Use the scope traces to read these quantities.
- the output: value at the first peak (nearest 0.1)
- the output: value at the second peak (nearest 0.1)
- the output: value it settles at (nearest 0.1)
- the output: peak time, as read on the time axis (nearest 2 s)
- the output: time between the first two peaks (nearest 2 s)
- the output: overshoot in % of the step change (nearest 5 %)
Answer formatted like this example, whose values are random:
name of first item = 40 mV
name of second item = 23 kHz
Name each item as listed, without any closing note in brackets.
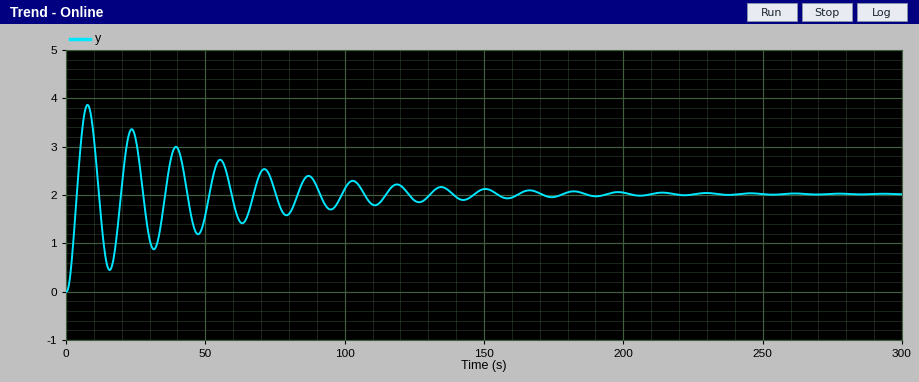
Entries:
the output: value at the first peak = 3.9
the output: value at the second peak = 3.4
the output: value it settles at = 2.0
the output: peak time, as read on the time axis = 8 s
the output: time between the first two peaks = 16 s
the output: overshoot in % of the step change = 90 %
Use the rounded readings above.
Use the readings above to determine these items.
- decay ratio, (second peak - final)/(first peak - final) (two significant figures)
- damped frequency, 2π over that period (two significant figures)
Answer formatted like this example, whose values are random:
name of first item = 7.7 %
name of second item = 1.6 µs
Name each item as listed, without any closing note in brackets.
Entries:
decay ratio, (second peak - final)/(first peak - final) = 0.74
damped frequency, 2π over that period = 0.39 rad/s
